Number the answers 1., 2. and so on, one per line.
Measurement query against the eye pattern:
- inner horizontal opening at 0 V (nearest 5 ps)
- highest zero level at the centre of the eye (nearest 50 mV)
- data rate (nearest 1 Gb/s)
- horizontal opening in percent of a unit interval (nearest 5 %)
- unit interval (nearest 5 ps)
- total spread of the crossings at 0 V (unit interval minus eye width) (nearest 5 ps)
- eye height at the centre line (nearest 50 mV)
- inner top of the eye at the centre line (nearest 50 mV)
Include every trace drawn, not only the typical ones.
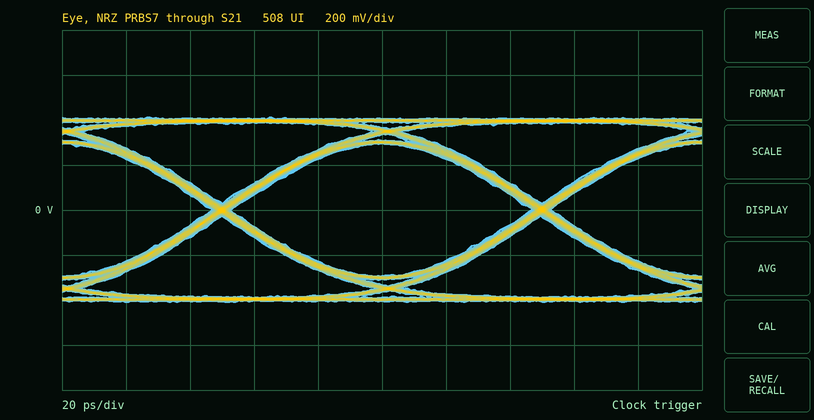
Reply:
1. 95 ps
2. -300 mV
3. 10 Gb/s
4. 95 %
5. 100 ps
6. 5 ps
7. 600 mV
8. 300 mV
